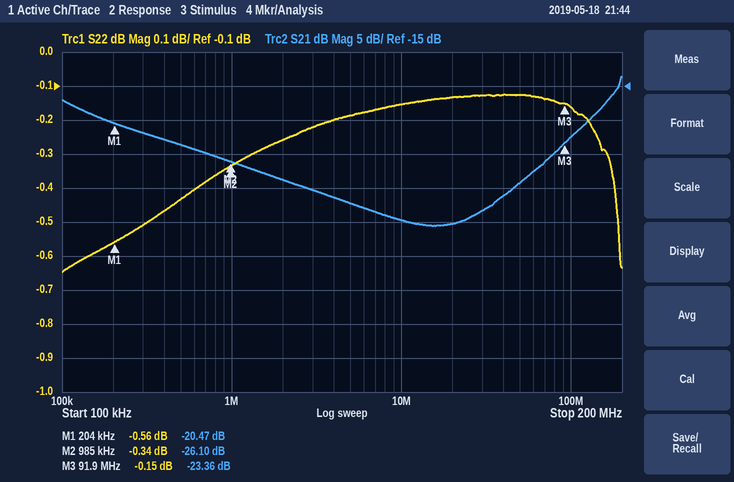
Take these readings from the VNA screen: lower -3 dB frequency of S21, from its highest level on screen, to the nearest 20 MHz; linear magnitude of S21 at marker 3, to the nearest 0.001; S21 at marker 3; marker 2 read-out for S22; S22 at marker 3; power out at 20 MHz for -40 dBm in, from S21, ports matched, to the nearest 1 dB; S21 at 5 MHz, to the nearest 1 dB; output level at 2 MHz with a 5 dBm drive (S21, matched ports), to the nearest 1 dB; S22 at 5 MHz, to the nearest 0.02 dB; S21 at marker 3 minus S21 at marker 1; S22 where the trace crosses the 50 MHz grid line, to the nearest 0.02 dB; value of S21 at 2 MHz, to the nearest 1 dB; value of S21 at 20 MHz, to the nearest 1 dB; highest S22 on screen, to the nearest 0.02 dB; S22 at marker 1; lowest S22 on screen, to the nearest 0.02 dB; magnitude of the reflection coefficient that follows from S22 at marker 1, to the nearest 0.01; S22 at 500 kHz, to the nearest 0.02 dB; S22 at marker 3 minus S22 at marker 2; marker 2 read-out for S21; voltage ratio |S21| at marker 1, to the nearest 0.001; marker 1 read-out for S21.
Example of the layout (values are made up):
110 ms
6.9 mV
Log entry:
180 MHz
0.068
-23.36 dB
-0.34 dB
-0.15 dB
-75 dBm
-32 dB
-24 dBm
-0.18 dB
-2.89 dB
-0.12 dB
-29 dB
-35 dB
-0.12 dB
-0.56 dB
-0.64 dB
0.94
-0.44 dB
0.19 dB
-26.10 dB
0.095
-20.47 dB
